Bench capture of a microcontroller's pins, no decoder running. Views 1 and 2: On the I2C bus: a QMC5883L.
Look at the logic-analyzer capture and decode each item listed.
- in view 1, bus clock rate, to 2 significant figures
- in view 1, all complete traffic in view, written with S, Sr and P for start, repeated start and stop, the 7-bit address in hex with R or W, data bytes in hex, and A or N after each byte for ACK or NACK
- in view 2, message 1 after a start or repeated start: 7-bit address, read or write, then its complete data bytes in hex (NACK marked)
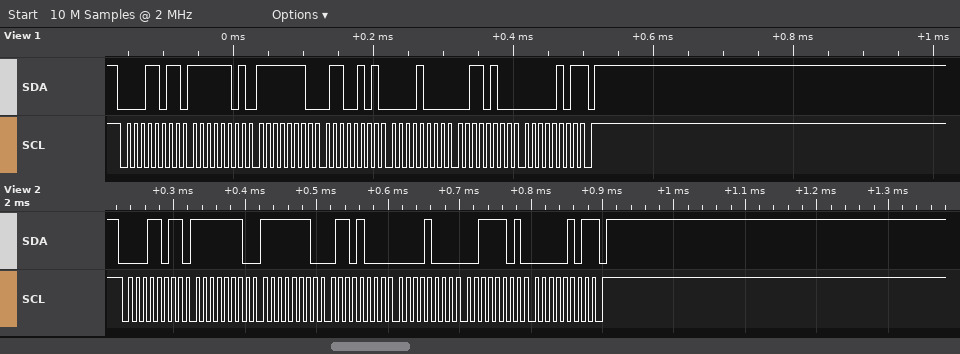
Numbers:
100 kHz
S 0DR A FD A FE A 65 A 08 A 34 A 05 N P
0x0D read: FE FE 68 08 3D 05 NACK
